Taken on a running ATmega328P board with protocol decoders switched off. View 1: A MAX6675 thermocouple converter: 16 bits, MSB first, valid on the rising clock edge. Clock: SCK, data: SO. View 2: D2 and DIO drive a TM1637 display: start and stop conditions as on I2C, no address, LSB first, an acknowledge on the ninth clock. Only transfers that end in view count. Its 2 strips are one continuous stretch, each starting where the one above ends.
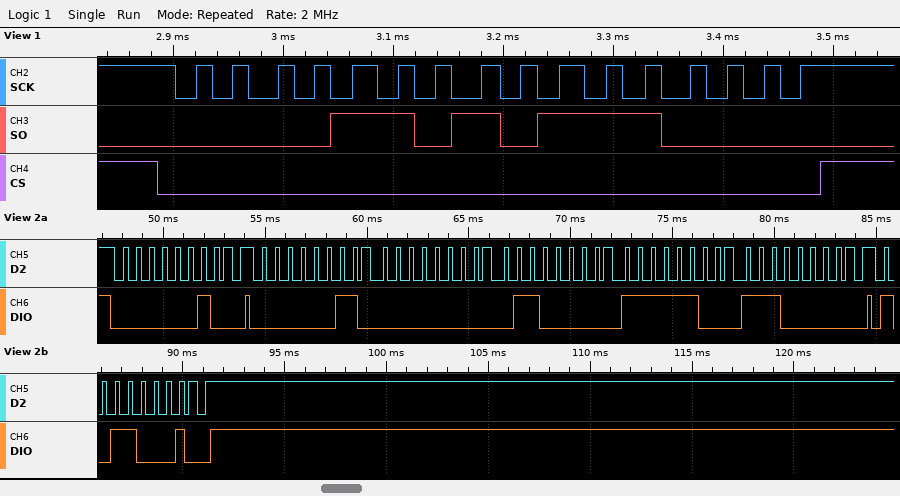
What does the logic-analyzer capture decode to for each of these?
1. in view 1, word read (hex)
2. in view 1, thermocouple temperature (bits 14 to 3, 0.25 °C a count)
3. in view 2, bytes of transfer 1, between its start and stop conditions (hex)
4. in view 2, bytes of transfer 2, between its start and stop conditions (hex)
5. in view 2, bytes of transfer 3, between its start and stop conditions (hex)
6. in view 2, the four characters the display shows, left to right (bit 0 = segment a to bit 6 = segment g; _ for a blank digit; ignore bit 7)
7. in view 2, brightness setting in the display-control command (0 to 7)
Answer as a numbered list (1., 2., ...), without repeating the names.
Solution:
1. 0x0D70
2. 107.50 °C
3. 40
4. C0 00 06 3F 07
5. 8D
6. _107
7. 5
